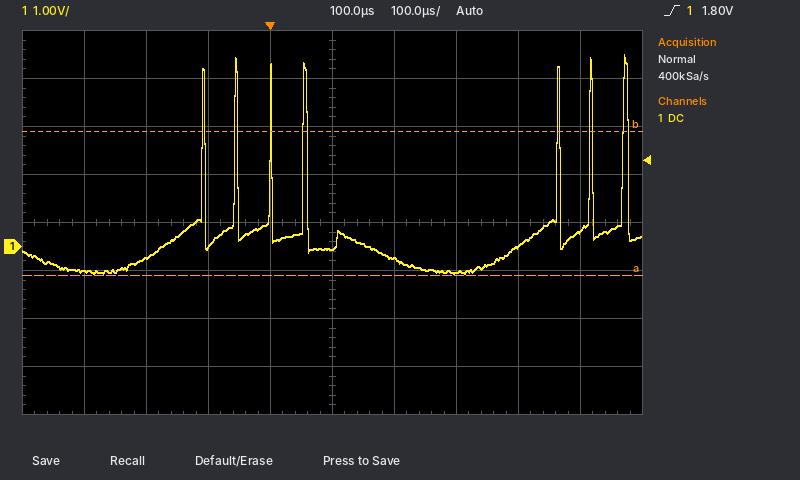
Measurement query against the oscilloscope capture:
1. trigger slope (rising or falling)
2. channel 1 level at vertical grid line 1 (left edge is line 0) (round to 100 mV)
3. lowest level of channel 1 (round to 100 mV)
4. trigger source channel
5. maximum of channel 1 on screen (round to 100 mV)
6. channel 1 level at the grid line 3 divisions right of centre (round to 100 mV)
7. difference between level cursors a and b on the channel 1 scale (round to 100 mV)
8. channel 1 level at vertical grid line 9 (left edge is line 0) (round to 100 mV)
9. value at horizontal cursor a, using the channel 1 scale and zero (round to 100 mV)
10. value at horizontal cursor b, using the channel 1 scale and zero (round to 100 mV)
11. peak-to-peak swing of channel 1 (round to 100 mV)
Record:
rising
-500 mV
-600 mV
channel 1
4.0 V
0.0 V
3.0 V
300 mV
-600 mV
2.4 V
4.6 V
